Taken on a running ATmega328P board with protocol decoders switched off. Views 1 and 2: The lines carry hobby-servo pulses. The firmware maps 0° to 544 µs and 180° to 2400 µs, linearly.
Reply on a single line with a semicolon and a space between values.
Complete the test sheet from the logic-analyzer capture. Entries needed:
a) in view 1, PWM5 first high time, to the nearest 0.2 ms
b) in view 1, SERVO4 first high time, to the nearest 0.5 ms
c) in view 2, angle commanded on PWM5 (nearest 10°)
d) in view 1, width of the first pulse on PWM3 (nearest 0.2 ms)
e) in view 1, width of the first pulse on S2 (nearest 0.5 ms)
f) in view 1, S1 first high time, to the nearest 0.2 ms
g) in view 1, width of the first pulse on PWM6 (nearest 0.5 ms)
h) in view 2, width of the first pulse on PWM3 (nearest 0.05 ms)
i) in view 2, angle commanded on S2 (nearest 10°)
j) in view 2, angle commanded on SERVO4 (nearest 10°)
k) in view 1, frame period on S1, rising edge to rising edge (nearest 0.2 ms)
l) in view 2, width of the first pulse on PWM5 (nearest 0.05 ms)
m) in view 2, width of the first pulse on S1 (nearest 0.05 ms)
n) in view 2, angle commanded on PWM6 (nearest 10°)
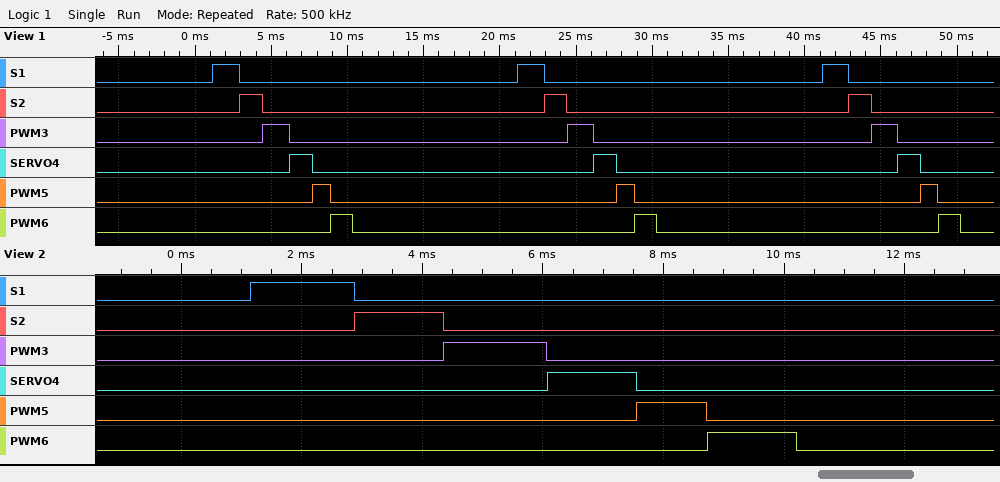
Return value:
1.2 ms; 1.5 ms; 60°; 1.8 ms; 1.5 ms; 1.8 ms; 1.5 ms; 1.70 ms; 90°; 90°; 20.0 ms; 1.15 ms; 1.70 ms; 90°
